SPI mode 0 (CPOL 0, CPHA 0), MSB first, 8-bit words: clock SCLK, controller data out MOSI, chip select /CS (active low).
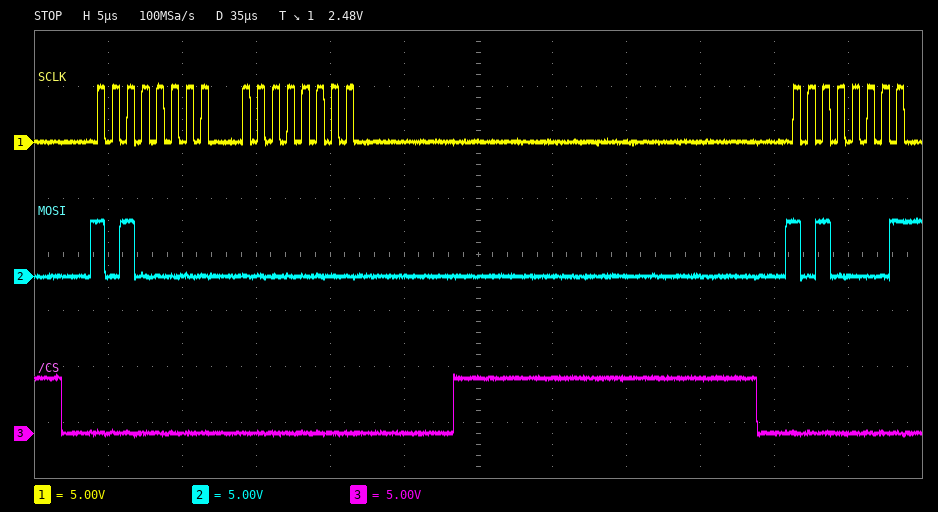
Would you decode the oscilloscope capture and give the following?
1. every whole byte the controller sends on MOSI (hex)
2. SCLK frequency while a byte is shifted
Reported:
A0 00 A1
1 MHz
